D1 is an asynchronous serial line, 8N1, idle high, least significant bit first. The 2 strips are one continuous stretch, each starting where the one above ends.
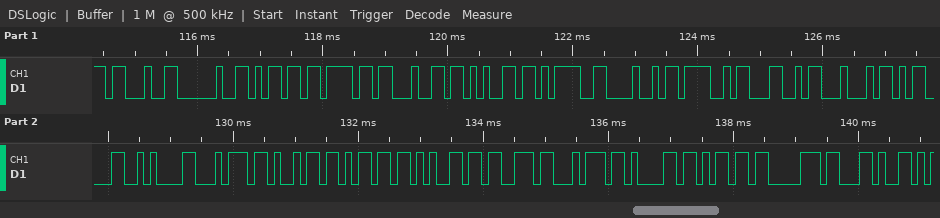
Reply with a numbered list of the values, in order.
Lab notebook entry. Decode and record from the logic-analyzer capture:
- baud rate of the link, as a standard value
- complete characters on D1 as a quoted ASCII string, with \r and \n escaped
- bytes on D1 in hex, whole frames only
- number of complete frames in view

1. 9600 baud
2. "# mode=HOLD\r\ntimestamp,"
3. 23 20 6D 6F 64 65 3D 48 4F 4C 44 0D 0A 74 69 6D 65 73 74 61 6D 70 2C
4. 23
